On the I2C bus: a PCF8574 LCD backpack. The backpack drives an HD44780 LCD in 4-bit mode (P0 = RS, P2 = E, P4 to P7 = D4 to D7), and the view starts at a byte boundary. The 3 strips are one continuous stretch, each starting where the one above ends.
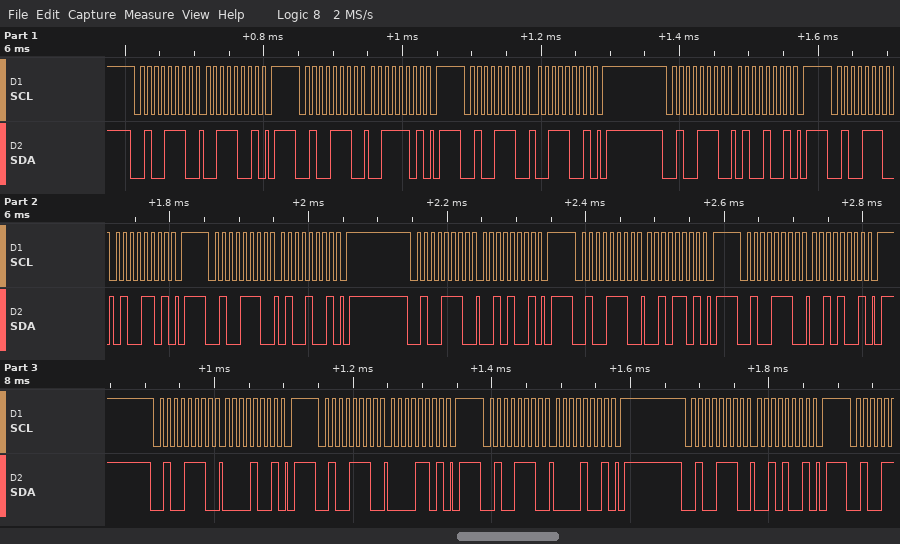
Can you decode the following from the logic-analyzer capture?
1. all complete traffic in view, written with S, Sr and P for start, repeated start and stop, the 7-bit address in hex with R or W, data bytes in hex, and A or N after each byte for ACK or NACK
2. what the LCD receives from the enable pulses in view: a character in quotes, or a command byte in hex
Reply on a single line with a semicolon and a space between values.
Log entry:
S 27W A 39 A P S 27W A 3D A P S 27W A 39 A P S 27W A 49 A P S 27W A 4D A P S 27W A 49 A P S 27W A 29 A P S 27W A 2D A P S 27W A 29 A P S 27W A 09 A P S 27W A 0D A P S 27W A 09 A P S 27W A 29 A P; '4' ' '
